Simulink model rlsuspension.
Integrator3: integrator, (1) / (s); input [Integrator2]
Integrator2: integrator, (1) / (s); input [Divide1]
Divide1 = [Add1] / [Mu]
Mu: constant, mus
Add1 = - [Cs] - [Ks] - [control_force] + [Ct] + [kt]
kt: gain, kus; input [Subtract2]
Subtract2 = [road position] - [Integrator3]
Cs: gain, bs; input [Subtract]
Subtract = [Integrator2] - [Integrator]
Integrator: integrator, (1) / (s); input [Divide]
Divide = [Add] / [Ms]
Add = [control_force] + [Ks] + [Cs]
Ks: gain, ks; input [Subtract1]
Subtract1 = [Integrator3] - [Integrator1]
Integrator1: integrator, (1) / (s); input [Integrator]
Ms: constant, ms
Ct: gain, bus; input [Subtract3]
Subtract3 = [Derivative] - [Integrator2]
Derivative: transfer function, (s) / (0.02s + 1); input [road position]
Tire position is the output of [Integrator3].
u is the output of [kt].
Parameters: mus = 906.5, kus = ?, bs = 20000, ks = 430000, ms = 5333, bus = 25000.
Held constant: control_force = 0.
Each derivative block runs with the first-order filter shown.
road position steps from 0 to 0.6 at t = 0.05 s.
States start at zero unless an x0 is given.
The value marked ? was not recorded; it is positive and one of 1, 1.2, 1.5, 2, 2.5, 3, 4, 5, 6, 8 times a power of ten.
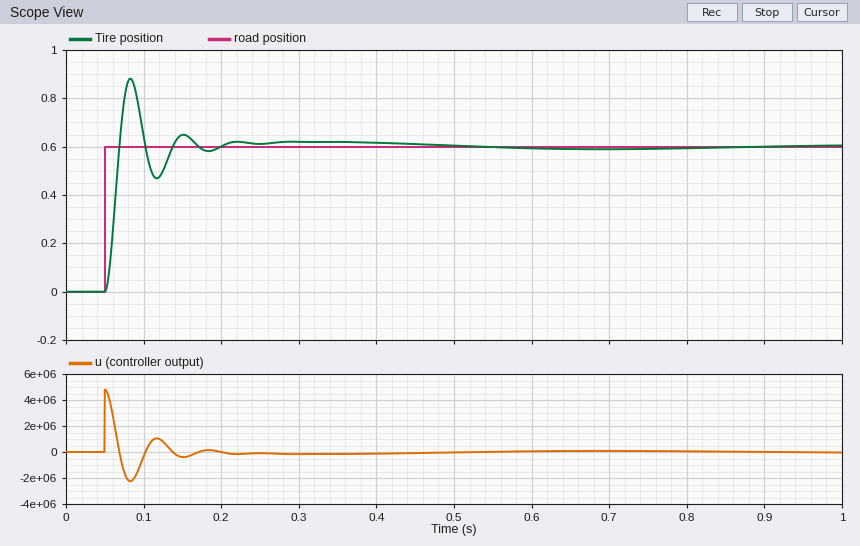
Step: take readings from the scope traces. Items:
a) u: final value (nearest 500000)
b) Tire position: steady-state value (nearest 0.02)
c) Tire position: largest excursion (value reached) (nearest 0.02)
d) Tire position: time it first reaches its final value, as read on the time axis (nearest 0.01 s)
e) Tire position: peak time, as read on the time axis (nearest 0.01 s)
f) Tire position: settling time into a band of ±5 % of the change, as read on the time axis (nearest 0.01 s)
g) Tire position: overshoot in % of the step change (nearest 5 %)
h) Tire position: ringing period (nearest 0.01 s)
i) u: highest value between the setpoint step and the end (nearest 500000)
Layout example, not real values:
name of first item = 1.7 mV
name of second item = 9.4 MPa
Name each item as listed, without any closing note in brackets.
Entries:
u: final value = 0
Tire position: steady-state value = 0.60
Tire position: largest excursion (value reached) = 0.88
Tire position: time it first reaches its final value, as read on the time axis = 0.07 s
Tire position: peak time, as read on the time axis = 0.08 s
Tire position: settling time into a band of ±5 % of the change, as read on the time axis = 0.16 s
Tire position: overshoot in % of the step change = 45 %
Tire position: ringing period = 0.07 s
u: highest value between the setpoint step and the end = 5000000
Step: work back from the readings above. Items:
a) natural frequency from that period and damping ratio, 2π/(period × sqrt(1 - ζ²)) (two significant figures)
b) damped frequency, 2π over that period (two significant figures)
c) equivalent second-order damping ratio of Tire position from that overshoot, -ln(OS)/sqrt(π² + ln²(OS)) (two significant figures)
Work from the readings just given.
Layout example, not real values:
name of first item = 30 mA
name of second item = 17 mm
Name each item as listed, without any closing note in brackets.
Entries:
natural frequency from that period and damping ratio, 2π/(period × sqrt(1 - ζ²)) = 93 rad/s
damped frequency, 2π over that period = 90 rad/s
equivalent second-order damping ratio of Tire position from that overshoot, -ln(OS)/sqrt(π² + ln²(OS)) = 0.25
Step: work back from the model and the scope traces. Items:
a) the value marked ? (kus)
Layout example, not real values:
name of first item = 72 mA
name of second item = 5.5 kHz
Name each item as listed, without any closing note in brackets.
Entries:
the value marked ? = 8e+06
